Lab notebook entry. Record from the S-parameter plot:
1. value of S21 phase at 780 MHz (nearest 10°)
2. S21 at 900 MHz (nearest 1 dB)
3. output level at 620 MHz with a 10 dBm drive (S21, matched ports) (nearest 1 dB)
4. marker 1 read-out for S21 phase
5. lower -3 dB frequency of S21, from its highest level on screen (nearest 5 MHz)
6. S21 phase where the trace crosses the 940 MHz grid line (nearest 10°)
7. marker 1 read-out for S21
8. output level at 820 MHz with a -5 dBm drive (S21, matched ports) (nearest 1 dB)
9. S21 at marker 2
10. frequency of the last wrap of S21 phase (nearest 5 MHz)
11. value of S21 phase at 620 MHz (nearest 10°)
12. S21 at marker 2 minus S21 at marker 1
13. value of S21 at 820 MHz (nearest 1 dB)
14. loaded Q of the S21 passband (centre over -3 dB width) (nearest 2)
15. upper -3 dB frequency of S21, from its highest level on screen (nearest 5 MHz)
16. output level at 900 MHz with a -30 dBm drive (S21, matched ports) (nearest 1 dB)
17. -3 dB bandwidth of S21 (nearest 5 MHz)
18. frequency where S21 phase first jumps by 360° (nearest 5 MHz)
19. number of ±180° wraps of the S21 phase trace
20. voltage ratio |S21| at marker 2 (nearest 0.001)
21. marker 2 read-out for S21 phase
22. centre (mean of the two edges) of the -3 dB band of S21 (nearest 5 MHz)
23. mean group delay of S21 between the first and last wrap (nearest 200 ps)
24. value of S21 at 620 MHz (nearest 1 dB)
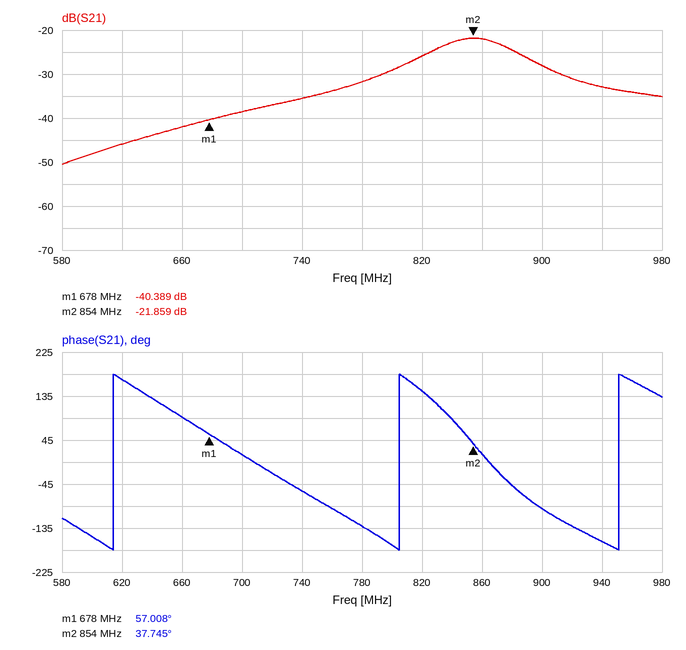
-130°
-28 dB
-36 dBm
57.008°
825 MHz
-160°
-40.389 dB
-31 dBm
-21.859 dB
950 MHz
170°
18.530 dB
-26 dB
16
880 MHz
-58 dBm
55 MHz
615 MHz
3
0.081
37.745°
855 MHz
6.0 ns
-46 dB
